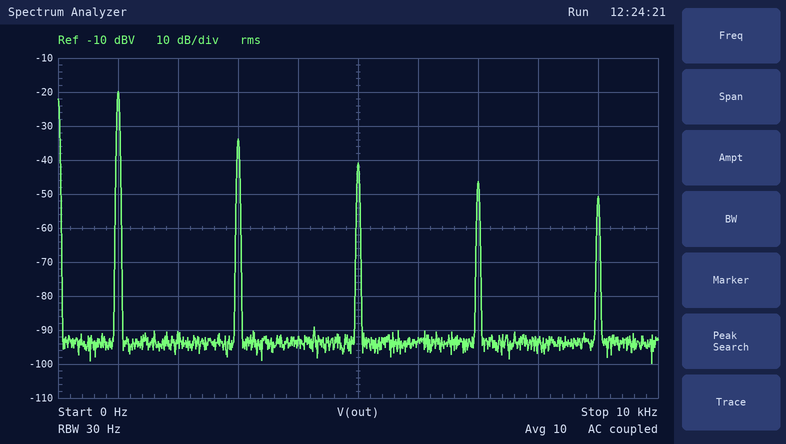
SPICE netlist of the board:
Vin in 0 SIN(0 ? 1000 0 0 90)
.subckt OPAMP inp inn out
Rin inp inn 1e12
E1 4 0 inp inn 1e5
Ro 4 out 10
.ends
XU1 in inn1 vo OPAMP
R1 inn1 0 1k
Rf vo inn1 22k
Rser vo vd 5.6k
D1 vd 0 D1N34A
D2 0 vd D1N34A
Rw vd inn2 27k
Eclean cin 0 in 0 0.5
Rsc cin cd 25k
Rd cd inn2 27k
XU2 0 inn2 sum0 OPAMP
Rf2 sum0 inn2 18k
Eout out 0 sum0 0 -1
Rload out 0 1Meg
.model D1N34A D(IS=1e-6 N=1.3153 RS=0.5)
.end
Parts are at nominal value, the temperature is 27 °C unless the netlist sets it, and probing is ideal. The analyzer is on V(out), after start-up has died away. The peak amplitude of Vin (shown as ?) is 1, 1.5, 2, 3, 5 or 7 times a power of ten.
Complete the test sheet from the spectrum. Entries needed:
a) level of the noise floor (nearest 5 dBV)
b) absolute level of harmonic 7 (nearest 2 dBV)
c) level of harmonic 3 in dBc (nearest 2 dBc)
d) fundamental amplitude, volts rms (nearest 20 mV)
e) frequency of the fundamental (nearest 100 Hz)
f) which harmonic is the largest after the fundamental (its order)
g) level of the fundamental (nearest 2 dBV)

-95 dBV
-46 dBV
-14 dBc
100 mV
1.0 kHz
3
-20 dBV
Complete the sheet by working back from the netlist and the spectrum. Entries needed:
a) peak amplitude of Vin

50 mV
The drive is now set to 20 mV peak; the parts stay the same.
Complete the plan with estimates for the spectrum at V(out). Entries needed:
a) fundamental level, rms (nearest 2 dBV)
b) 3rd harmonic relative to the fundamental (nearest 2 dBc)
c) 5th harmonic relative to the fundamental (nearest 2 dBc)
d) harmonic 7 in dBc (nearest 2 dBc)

-22 dBV
-16 dBc
-26 dBc
-36 dBc
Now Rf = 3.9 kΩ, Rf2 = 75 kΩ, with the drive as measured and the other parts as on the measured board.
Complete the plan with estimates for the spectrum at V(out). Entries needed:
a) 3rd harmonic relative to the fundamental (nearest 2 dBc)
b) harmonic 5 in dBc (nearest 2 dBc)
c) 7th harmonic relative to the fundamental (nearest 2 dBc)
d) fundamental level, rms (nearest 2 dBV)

-22 dBc
-36 dBc
-50 dBc
-12 dBV
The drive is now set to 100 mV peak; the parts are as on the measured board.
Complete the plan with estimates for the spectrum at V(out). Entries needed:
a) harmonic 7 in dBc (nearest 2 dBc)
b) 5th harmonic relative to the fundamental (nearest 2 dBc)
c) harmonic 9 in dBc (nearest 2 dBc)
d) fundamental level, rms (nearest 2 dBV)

-24 dBc
-20 dBc
-28 dBc
-18 dBV
